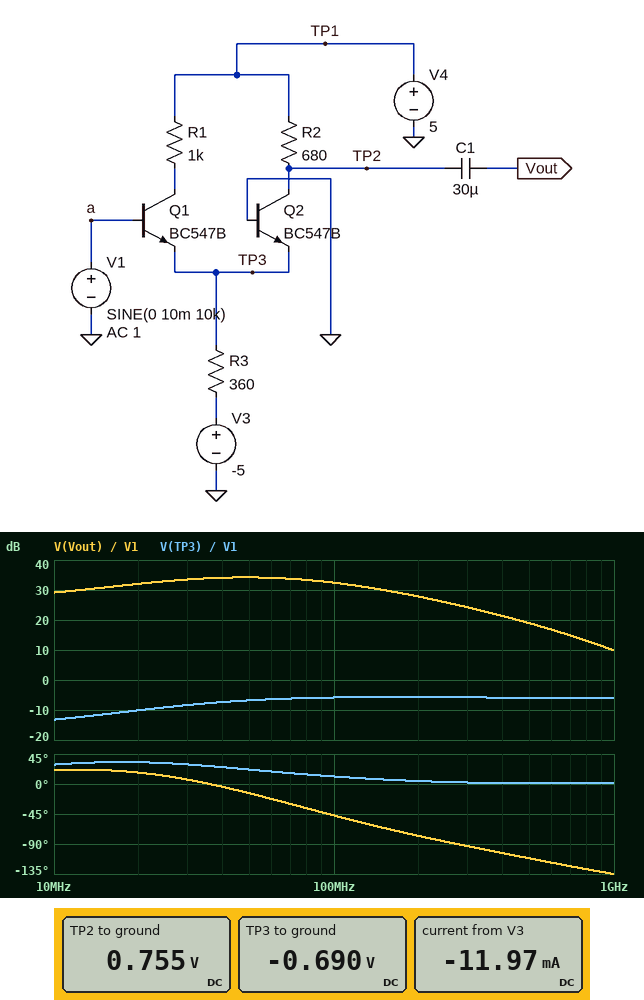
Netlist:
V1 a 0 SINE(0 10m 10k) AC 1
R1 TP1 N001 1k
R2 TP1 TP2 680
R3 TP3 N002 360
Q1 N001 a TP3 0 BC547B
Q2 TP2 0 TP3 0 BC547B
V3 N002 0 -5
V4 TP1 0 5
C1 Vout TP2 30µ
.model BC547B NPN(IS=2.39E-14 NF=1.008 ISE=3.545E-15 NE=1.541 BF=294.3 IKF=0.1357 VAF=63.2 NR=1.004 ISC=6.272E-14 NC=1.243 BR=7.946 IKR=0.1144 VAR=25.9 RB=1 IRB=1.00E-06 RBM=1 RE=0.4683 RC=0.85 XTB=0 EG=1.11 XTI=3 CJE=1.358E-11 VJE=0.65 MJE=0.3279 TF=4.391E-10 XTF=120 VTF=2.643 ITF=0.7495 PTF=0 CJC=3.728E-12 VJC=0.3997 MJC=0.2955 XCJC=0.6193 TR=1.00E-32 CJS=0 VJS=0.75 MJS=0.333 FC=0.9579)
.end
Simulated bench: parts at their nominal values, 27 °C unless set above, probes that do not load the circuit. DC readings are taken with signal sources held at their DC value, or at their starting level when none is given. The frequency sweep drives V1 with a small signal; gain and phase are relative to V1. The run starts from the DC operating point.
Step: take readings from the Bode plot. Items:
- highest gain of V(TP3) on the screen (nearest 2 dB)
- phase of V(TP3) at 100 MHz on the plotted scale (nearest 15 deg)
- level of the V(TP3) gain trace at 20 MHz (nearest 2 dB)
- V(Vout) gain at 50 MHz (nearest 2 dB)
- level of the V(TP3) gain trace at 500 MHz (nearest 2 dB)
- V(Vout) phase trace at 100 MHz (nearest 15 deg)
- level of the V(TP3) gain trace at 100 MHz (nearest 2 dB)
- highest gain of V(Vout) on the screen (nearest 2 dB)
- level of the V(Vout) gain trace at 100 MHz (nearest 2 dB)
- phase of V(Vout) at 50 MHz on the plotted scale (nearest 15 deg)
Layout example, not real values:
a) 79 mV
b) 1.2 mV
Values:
a) -6 dB
b) 15 deg
c) -10 dB
d) 34 dB
e) -6 dB
f) -45 deg
g) -6 dB
h) 34 dB
i) 32 dB
j) -15 deg
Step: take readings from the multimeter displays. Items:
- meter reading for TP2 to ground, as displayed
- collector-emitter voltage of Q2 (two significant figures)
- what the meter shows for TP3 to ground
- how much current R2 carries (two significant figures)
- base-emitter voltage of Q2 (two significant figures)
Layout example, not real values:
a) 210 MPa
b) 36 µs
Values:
a) 0.755 V
b) 1.4 V
c) -0.690 V
d) 6.2 mA
e) 690 mV
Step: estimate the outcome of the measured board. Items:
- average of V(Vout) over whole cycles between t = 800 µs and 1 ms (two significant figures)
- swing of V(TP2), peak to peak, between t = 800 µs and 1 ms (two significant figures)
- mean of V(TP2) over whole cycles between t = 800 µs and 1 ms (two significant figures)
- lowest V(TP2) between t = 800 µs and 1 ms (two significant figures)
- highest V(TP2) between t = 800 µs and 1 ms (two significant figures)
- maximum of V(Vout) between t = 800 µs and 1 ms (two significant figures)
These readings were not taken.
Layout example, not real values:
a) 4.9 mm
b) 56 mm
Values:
a) -72 mV
b) 690 mV
c) 680 mV
d) 270 mV
e) 960 mV
f) 210 mV
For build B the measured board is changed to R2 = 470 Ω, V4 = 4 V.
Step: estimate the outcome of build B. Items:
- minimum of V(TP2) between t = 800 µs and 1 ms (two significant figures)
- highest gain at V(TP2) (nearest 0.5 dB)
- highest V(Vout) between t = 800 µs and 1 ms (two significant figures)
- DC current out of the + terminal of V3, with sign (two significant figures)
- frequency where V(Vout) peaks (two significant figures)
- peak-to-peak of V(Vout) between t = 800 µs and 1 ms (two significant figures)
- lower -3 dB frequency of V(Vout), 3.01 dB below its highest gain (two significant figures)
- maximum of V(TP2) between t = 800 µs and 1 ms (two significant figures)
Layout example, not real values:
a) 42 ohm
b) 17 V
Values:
a) 600 mV
b) 31.0 dB
c) 150 mV
d) -12 mA
e) 86 MHz
f) 280 mV
g) 32 MHz
h) 880 mV
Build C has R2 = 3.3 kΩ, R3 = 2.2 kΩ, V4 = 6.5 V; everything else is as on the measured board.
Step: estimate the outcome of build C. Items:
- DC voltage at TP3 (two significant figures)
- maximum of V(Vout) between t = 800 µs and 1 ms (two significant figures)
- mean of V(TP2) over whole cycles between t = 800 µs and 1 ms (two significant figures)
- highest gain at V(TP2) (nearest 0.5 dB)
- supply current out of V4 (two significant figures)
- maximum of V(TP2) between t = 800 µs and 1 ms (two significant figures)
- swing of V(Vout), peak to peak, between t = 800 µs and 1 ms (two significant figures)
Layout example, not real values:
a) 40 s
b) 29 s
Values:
a) -640 mV
b) 580 mV
c) 3.3 V
d) 35.5 dB
e) 2.0 mA
f) 3.9 V
g) 1.2 V
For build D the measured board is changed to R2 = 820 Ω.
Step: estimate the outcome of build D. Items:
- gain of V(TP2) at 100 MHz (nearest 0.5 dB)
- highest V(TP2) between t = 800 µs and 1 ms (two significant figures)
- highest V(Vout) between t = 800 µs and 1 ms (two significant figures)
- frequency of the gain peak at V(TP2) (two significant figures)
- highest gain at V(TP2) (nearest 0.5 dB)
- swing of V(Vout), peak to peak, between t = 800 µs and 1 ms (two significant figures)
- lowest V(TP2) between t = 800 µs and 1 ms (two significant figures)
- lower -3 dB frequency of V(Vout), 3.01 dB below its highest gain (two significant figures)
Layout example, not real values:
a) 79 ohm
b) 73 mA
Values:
a) 30.5 dB
b) 140 mV
c) 250 mV
d) 37 MHz
e) 34.0 dB
f) 730 mV
g) -590 mV
h) 12 MHz
